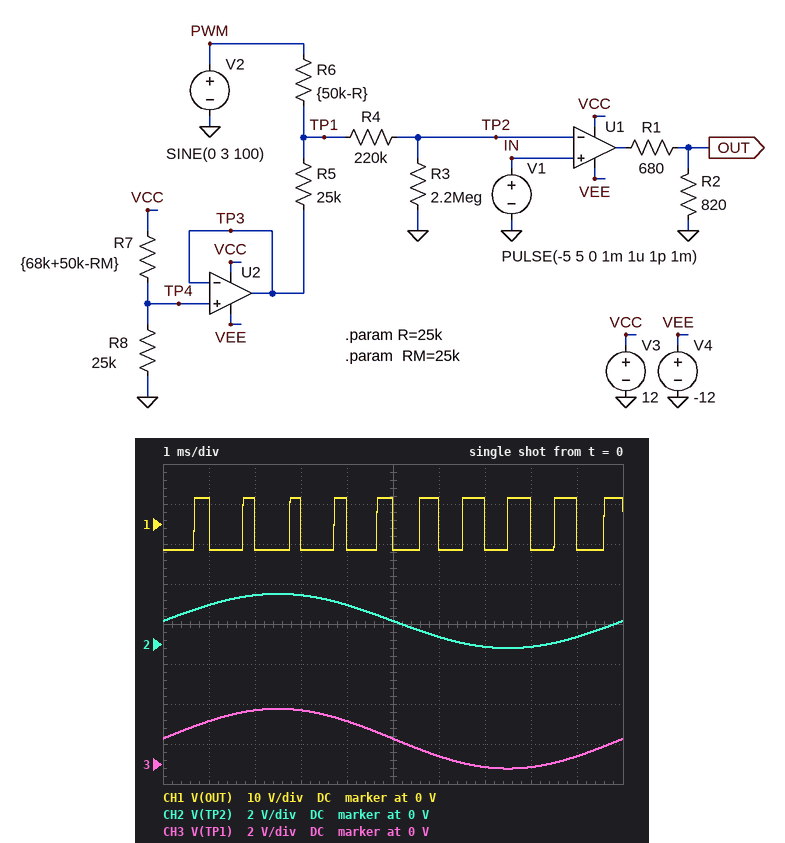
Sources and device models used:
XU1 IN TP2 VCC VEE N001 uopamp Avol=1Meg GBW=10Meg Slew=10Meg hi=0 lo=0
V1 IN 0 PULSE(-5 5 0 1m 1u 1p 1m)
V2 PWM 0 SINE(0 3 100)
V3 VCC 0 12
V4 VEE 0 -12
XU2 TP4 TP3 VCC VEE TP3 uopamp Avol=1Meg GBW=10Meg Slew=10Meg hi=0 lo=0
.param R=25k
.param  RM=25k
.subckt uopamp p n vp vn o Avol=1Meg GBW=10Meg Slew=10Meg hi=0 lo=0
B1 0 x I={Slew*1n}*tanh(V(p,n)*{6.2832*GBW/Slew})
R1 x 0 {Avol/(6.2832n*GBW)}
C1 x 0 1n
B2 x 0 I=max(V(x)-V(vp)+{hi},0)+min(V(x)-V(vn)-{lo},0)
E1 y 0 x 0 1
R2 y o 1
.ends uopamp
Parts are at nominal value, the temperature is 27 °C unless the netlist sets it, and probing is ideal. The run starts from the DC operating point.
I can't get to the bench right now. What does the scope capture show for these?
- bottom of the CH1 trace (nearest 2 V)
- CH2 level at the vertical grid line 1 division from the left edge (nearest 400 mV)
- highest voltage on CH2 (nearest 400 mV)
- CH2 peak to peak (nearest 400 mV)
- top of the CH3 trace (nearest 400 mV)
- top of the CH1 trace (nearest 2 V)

-6 V
2.0 V
2.4 V
2.8 V
2.8 V
6 V
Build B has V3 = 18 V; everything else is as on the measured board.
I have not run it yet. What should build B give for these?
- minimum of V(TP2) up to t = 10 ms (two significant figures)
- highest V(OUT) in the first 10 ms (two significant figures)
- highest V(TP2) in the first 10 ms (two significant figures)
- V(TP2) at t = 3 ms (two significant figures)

370 mV
9.8 V
3.1 V
3.0 V
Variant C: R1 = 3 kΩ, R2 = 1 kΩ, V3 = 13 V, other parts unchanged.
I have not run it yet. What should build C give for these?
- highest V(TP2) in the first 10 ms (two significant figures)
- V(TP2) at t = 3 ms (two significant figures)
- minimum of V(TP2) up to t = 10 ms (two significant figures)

2.6 V
2.5 V
-110 mV
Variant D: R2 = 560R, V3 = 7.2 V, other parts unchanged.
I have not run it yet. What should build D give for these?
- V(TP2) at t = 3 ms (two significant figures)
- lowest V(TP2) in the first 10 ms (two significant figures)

2.0 V
-670 mV
